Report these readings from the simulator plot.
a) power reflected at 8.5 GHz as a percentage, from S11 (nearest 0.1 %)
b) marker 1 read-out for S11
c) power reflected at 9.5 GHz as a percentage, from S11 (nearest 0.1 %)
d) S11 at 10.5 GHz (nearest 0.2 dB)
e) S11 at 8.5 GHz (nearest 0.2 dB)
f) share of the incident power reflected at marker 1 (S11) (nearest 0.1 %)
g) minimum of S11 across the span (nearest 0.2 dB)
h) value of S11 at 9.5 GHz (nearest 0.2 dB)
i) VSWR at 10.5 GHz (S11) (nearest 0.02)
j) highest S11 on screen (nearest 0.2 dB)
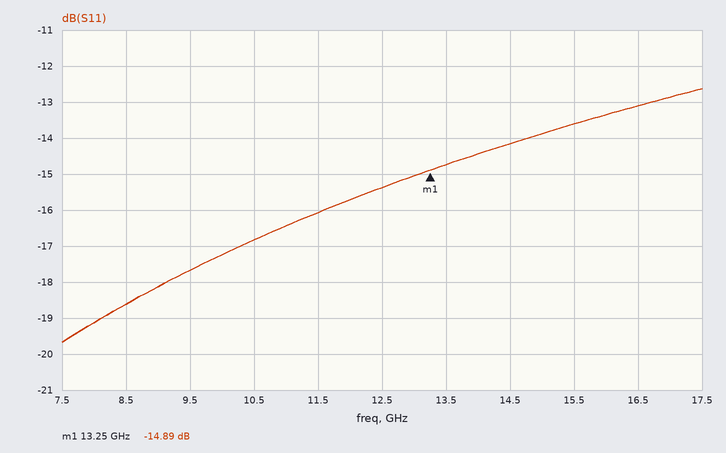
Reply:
1.4 %
-14.89 dB
1.7 %
-16.8 dB
-18.6 dB
3.2 %
-19.6 dB
-17.6 dB
1.34
-12.6 dB
